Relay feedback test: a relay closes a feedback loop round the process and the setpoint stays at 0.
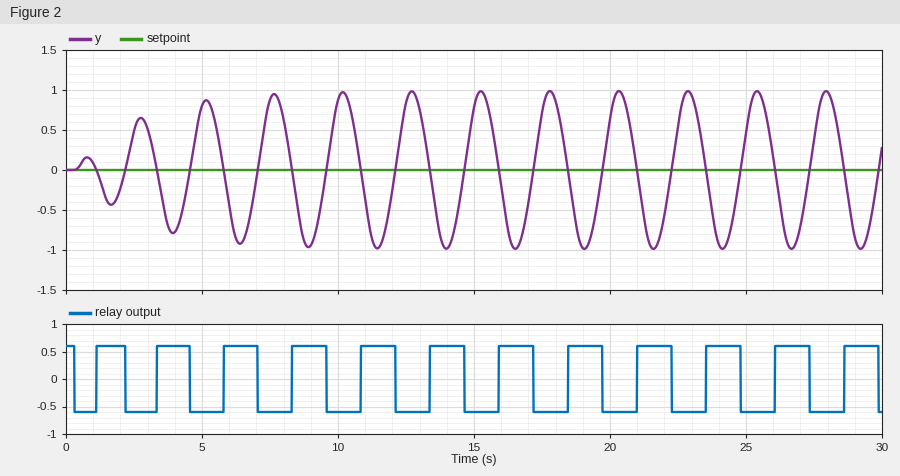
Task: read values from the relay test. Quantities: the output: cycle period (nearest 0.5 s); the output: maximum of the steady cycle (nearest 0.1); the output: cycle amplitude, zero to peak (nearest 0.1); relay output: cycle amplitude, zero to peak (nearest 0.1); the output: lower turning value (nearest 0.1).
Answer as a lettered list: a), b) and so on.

a) 2.5 s
b) 1.0
c) 1.0
d) 0.6
e) -1.0
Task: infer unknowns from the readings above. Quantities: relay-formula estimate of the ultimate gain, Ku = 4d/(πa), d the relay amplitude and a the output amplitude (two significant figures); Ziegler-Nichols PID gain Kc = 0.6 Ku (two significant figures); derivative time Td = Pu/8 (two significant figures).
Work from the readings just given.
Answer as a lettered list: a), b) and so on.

a) 0.76
b) 0.46
c) 0.31 s
